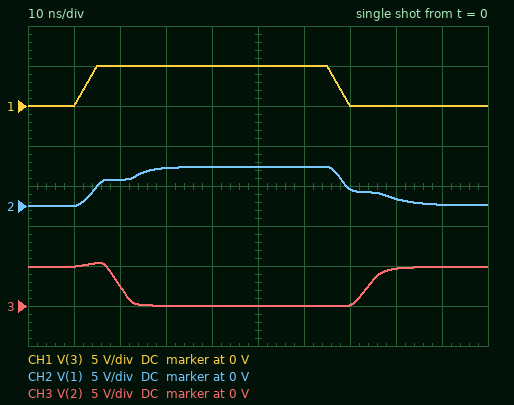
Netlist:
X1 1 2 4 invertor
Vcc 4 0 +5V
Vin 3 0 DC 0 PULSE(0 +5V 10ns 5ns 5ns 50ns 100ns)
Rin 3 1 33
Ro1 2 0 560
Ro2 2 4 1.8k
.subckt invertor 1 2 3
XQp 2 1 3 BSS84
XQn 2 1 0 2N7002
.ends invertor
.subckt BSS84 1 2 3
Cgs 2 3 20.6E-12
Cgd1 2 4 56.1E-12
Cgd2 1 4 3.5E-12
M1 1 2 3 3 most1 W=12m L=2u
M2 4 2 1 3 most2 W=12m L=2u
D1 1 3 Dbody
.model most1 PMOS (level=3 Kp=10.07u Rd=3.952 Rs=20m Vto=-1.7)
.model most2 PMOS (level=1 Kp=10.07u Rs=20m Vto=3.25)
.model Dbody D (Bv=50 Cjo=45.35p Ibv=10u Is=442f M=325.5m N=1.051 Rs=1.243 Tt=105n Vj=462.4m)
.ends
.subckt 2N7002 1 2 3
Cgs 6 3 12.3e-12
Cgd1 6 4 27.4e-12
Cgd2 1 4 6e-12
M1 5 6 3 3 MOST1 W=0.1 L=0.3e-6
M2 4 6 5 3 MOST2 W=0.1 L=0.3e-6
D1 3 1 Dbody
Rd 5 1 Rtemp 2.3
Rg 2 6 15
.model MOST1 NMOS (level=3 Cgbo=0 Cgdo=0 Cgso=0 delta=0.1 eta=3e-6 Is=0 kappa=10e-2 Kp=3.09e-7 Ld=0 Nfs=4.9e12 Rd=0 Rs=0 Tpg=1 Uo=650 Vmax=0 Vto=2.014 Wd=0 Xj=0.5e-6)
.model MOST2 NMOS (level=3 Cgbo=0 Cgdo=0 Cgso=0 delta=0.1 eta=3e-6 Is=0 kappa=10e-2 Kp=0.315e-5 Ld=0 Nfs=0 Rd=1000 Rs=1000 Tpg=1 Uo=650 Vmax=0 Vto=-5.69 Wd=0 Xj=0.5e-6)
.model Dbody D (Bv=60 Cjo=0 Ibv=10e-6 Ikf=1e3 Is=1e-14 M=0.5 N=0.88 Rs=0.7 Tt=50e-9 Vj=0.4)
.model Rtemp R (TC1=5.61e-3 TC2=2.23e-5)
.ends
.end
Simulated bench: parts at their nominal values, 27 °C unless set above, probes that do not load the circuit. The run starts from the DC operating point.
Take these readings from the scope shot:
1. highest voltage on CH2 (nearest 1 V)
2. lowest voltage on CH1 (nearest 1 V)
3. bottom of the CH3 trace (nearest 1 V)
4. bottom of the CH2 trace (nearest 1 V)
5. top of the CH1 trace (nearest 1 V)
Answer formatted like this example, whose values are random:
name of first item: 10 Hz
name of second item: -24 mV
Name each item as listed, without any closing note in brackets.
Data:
highest voltage on CH2: 5 V
lowest voltage on CH1: 0 V
bottom of the CH3 trace: 0 V
bottom of the CH2 trace: 0 V
top of the CH1 trace: 5 V
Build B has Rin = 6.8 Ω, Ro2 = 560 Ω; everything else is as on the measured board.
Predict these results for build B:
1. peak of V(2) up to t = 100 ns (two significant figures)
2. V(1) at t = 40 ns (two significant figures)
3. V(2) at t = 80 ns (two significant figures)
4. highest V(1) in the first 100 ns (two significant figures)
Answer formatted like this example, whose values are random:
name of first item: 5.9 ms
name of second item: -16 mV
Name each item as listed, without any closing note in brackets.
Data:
peak of V(2) up to t = 100 ns: 5.5 V
V(1) at t = 40 ns: 5.0 V
V(2) at t = 80 ns: 4.9 V
highest V(1) in the first 100 ns: 5.0 V
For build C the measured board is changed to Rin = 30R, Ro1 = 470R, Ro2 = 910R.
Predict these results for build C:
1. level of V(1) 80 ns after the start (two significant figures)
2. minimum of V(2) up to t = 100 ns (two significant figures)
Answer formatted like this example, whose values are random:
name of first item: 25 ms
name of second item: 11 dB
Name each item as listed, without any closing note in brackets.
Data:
level of V(1) 80 ns after the start: 720 mV
minimum of V(2) up to t = 100 ns: -21 mV
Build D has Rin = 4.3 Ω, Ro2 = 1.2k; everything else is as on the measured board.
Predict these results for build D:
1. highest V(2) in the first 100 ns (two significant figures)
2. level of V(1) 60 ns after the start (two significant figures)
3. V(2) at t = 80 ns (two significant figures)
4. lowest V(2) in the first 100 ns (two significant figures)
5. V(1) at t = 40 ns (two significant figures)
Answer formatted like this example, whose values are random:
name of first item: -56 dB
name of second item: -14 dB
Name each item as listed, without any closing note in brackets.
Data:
highest V(2) in the first 100 ns: 5.5 V
level of V(1) 60 ns after the start: 5.0 V
V(2) at t = 80 ns: 4.9 V
lowest V(2) in the first 100 ns: -47 mV
V(1) at t = 40 ns: 5.0 V
